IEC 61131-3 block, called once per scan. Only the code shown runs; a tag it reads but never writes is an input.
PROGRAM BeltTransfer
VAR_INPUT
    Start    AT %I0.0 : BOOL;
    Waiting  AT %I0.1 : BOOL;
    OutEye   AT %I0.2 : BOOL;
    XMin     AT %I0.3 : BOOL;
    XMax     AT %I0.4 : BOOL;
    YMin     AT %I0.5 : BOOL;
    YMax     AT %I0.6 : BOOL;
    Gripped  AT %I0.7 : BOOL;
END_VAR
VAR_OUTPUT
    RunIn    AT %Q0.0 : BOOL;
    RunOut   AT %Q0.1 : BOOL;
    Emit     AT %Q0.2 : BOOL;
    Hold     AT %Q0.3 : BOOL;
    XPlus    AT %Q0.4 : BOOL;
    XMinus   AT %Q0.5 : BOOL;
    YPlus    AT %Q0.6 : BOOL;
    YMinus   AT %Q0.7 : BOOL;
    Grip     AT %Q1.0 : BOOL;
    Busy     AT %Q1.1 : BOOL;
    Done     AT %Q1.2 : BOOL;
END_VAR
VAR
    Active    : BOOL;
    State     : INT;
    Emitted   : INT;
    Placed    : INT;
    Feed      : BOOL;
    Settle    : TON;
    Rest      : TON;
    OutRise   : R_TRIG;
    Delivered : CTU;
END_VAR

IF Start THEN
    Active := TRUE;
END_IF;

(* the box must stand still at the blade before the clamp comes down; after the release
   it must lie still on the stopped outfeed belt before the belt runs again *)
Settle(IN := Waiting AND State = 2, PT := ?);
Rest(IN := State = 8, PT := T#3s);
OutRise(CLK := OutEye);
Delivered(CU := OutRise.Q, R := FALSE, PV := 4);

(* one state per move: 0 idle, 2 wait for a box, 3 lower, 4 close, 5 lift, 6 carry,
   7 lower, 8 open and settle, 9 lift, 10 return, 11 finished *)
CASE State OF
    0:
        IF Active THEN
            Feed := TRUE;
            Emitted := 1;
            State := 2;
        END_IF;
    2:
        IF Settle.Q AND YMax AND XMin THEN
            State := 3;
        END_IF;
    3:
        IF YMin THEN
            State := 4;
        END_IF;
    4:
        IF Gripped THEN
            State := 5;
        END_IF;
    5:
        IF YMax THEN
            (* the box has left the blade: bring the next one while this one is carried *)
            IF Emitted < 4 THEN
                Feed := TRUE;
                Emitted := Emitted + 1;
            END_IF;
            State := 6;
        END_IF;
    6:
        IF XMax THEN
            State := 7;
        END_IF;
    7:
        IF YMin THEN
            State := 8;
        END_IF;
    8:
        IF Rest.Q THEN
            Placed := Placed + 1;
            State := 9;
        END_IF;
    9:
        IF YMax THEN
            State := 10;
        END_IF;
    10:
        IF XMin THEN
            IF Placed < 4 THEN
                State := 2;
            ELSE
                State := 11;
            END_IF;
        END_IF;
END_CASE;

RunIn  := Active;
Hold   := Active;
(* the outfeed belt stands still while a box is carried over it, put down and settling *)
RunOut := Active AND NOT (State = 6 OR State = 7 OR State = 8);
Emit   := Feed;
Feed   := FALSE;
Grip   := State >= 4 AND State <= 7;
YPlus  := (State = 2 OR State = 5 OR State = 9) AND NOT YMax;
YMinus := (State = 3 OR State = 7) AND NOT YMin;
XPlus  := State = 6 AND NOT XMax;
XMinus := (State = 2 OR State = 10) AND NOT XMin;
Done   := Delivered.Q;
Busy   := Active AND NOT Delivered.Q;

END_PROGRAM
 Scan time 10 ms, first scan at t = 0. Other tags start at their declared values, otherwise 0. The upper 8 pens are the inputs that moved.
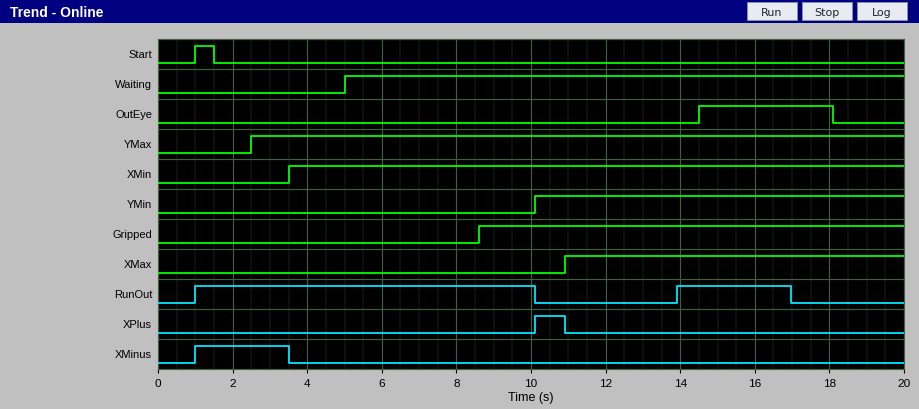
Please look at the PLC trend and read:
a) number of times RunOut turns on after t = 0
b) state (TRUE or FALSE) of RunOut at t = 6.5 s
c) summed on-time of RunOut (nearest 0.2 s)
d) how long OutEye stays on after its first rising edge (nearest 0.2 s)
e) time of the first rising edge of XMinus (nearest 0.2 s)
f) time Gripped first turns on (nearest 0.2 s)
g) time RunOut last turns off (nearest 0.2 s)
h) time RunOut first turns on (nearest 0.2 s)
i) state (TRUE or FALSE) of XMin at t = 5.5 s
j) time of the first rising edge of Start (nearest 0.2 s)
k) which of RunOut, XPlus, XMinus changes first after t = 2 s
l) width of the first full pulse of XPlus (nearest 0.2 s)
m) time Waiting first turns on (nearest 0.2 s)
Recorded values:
2
TRUE
12.2 s
3.6 s
1.0 s
8.6 s
17.0 s
1.0 s
TRUE
1.0 s
XMinus
0.8 s
5.0 s
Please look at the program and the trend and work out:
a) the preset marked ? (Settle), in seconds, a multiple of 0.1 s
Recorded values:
3.0 s
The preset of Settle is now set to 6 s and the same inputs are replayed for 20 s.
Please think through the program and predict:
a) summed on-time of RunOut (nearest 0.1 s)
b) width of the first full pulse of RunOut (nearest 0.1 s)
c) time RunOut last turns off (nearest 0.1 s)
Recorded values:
16.0 s
10.0 s
11.0 s
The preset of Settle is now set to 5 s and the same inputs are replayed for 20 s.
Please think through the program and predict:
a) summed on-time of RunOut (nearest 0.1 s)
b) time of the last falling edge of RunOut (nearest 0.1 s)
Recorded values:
14.2 s
19.0 s
